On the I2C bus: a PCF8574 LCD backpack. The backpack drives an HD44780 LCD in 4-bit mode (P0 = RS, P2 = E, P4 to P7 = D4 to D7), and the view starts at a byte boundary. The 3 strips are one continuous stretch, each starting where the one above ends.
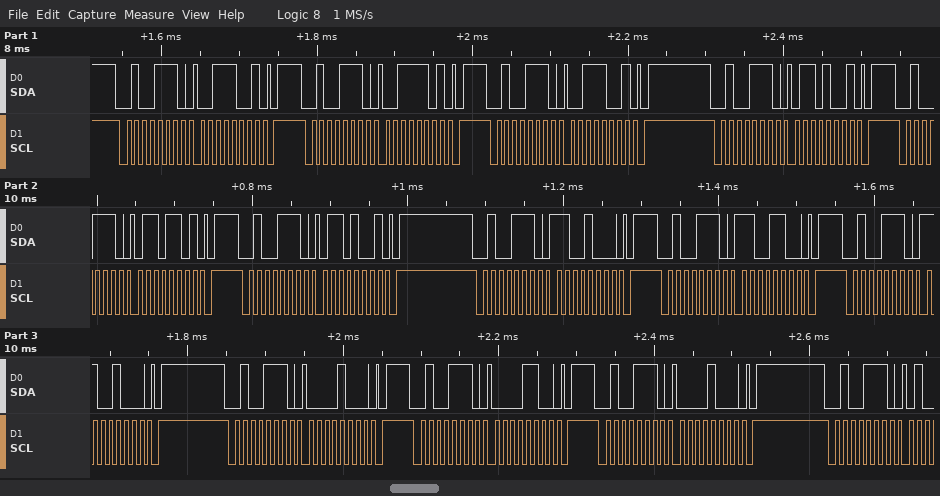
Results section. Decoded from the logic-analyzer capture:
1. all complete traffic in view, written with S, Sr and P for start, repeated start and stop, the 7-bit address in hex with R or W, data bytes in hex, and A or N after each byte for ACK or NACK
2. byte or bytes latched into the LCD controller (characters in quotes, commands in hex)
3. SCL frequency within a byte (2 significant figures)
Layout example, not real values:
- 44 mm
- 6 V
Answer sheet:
- S 27W A 39 A P S 27W A 3D A P S 27W A 39 A P S 27W A 69 A P S 27W A 6D A P S 27W A 69 A P S 27W A C8 A P S 27W A CC A P S 27W A C8 A P S 27W A 08 A P S 27W A 0C A P S 27W A 08 A P S 27W A
- '6' 0xC0
- 100 kHz
